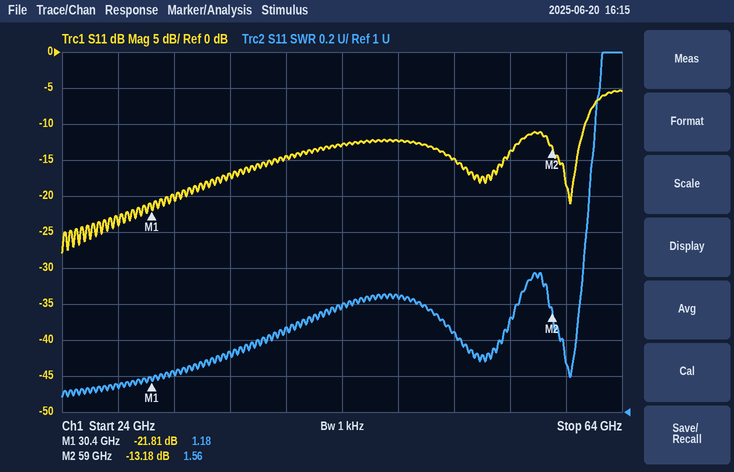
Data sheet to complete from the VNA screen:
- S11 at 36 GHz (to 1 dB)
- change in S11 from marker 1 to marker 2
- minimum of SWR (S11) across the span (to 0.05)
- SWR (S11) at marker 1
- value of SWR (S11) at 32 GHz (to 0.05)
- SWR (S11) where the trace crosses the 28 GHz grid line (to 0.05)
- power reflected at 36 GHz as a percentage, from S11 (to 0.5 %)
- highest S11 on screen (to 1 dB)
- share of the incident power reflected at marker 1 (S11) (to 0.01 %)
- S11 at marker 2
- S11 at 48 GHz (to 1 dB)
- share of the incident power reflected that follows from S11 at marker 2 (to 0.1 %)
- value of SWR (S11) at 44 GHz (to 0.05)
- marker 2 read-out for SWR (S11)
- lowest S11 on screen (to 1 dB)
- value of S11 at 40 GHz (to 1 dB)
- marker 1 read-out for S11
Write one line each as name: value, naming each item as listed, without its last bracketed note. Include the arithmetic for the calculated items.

S11 at 36 GHz: -17 dB
change in S11 from marker 1 to marker 2: -13.18 − (-21.81) = 8.63 dB
minimum of SWR (S11) across the span: 1.10
SWR (S11) at marker 1: 1.18
value of SWR (S11) at 32 GHz: 1.20
SWR (S11) where the trace crosses the 28 GHz grid line: 1.15
power reflected at 36 GHz as a percentage, from S11: 10^(-17/10) ≈ 2.0 %
highest S11 on screen: -5 dB
share of the incident power reflected at marker 1 (S11): 10^(-21.81/10) ≈ 0.66 %
S11 at marker 2: -13.18 dB
S11 at 48 GHz: -12 dB
share of the incident power reflected that follows from S11 at marker 2: 10^(-13.18/10) ≈ 4.8 %
value of SWR (S11) at 44 GHz: 1.60
marker 2 read-out for SWR: 1.56
lowest S11 on screen: -28 dB
value of S11 at 40 GHz: -14 dB
marker 1 read-out for S11: -21.81 dB
